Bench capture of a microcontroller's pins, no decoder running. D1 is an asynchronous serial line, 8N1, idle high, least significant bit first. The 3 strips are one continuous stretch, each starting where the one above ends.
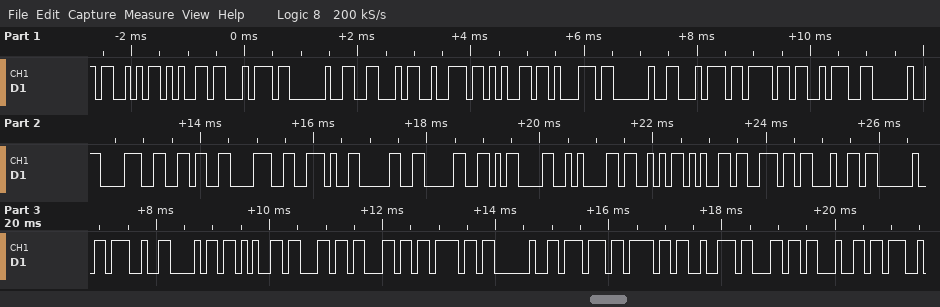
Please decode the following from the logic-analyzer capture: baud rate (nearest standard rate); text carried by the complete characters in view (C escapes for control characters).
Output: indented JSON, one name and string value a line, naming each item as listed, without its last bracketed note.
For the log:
{
  "baud rate": "9600 baud",
  "text carried by the complete characters in view": "\"Set Freq to: 868.00\\r\\nSend 'hello world\""
}
